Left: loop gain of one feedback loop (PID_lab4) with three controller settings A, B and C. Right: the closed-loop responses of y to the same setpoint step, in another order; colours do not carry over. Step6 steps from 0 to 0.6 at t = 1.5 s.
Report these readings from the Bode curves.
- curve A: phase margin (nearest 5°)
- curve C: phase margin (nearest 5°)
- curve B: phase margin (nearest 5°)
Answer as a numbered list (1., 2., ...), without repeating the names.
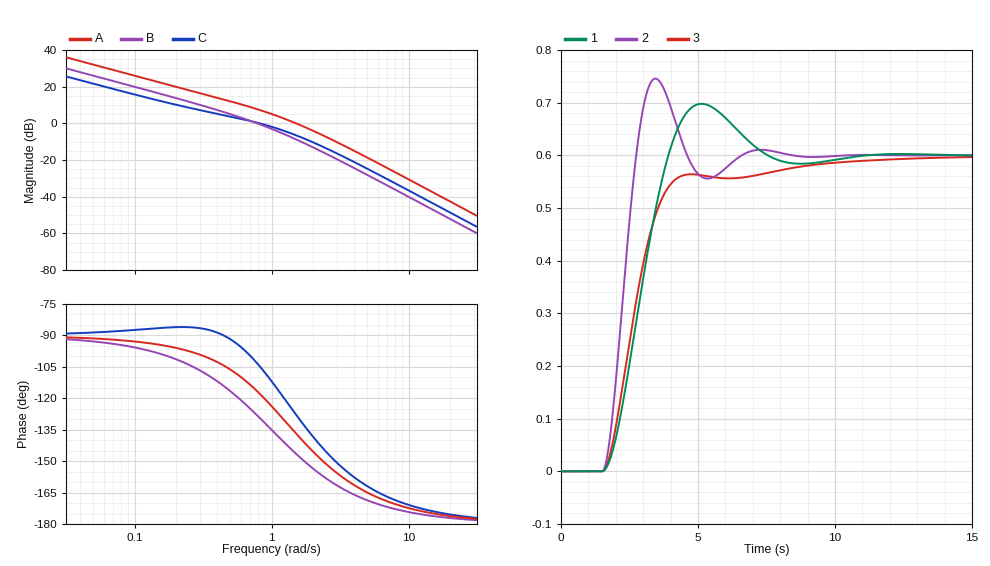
1. 45°
2. 75°
3. 50°
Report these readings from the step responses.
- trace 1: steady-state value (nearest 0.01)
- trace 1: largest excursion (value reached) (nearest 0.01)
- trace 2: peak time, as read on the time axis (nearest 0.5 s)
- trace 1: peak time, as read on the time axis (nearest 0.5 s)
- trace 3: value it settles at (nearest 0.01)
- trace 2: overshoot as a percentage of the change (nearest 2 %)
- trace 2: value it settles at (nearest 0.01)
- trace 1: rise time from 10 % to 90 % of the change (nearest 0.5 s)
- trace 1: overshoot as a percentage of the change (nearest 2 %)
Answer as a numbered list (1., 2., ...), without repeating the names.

1. 0.60
2. 0.70
3. 3.5 s
4. 5.0 s
5. 0.60
6. 24 %
7. 0.60
8. 1.5 s
9. 16 %
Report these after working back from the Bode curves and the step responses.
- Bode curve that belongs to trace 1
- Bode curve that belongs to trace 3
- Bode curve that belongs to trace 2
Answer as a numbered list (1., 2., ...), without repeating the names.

1. B
2. C
3. A
